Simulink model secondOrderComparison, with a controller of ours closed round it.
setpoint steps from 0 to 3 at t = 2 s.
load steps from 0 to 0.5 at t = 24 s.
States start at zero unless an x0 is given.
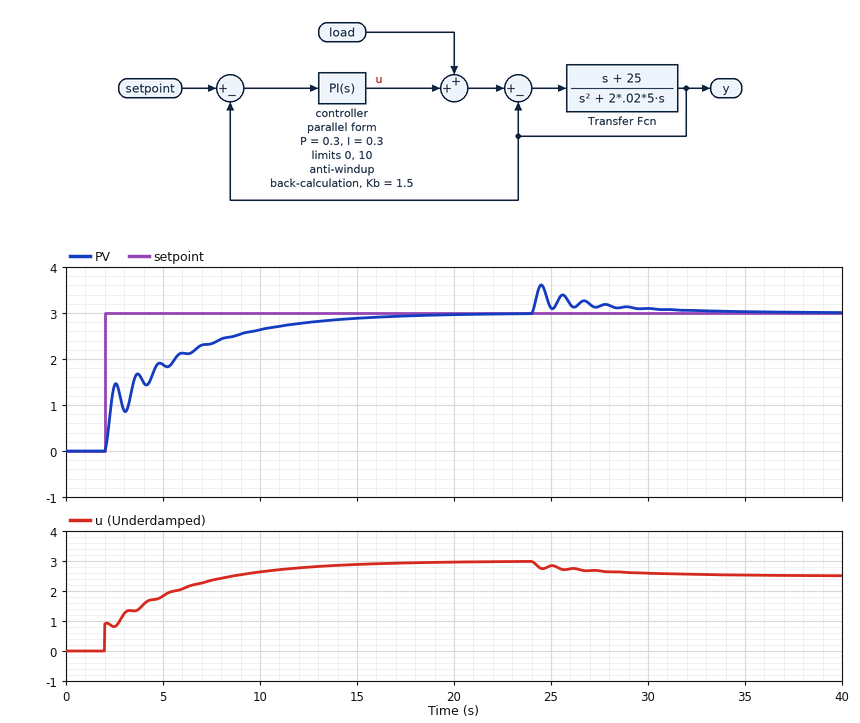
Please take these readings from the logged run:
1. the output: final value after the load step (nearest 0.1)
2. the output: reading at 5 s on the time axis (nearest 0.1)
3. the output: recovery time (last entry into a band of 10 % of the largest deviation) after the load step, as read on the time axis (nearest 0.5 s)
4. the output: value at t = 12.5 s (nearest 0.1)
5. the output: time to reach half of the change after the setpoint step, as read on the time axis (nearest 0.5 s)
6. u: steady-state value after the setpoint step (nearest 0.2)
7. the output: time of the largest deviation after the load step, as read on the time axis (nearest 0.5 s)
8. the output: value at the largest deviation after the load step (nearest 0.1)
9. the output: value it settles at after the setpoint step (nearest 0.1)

3.0
1.9
31.5 s
2.8
3.5 s
3.0
24.5 s
3.6
3.0
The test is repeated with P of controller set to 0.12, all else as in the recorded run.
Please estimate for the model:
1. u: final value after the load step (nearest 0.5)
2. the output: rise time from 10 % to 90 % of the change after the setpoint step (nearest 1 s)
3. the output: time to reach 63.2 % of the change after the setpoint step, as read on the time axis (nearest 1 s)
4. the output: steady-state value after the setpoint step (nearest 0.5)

2.5
8 s
5 s
3.0
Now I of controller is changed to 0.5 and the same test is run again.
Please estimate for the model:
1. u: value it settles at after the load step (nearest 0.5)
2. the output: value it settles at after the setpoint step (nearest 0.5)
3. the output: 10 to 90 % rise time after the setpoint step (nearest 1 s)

2.5
3.0
5 s
